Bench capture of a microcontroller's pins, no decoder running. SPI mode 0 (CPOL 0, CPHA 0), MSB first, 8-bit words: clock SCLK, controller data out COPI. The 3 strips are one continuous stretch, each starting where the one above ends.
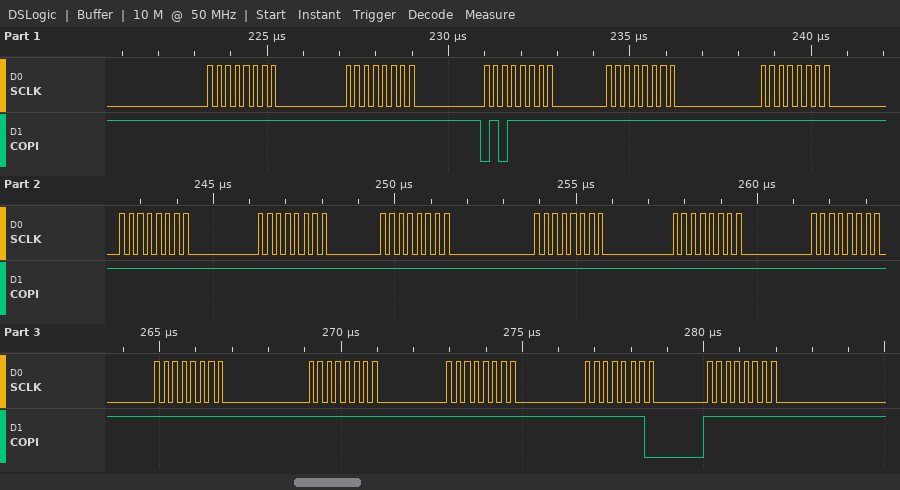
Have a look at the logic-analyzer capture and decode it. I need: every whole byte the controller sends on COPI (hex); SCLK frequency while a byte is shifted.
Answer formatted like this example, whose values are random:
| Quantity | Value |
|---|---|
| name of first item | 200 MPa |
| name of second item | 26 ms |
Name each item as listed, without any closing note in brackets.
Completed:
| Quantity | Value |
|---|---|
| every whole byte the controller sends on COPI | FF FF 5F FF FF FF FF FF FF FF FF FF FF FF FE FF |
| SCLK frequency while a byte is shifted | 4 MHz |
